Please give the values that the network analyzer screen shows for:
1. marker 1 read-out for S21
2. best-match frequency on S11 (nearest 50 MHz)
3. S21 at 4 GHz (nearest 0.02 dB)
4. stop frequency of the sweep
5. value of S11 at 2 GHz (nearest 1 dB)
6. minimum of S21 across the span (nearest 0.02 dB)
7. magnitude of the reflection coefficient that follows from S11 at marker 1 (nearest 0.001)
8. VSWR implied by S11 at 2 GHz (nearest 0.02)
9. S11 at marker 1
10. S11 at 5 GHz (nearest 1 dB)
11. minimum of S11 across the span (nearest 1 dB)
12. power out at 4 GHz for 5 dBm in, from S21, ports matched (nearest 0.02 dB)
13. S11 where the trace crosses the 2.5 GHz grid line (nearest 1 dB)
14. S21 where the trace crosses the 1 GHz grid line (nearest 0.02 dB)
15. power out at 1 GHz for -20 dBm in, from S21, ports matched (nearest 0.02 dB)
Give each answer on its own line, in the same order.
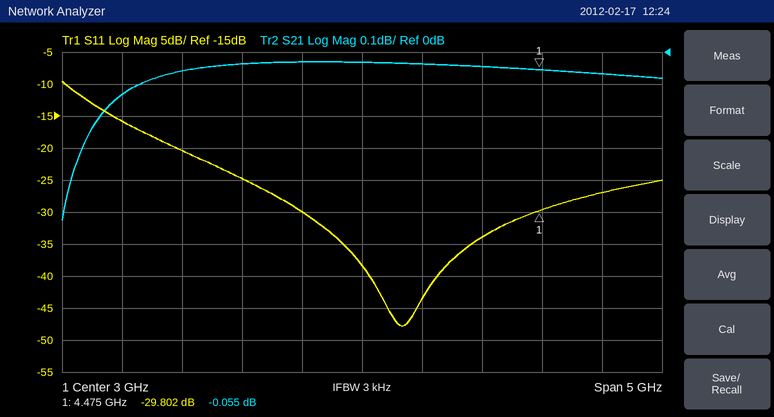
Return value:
-0.055 dB
3.35 GHz
-0.04 dB
5.5 GHz
-25 dB
-0.52 dB
0.032
1.12
-29.802 dB
-27 dB
-48 dB
4.96 dBm
-30 dB
-0.14 dB
-20.14 dBm
